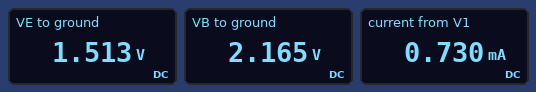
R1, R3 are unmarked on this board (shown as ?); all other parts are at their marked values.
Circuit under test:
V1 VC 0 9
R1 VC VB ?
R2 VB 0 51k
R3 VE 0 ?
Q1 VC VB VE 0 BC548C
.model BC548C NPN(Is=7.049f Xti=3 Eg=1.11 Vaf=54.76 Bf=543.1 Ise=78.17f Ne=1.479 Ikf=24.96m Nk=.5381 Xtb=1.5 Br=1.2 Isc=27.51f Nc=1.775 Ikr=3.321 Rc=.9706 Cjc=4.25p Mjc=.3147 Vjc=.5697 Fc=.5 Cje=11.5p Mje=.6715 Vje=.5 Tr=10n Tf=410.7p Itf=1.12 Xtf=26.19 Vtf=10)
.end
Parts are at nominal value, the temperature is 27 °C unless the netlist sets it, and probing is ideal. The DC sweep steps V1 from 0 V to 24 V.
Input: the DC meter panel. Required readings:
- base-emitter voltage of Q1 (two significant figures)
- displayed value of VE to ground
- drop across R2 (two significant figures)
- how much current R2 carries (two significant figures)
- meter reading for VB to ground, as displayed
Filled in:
650 mV
1.513 V
2.2 V
42 µA
2.165 V
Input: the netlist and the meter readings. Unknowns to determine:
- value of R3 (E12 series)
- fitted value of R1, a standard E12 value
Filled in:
2.2 kΩ
150 kΩ
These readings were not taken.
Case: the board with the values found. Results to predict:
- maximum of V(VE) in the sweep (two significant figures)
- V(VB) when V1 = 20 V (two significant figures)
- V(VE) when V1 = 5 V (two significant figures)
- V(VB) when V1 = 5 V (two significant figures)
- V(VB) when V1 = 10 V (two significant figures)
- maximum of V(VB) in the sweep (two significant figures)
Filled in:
5.1 V
4.8 V
580 mV
1.2 V
2.4 V
5.8 V
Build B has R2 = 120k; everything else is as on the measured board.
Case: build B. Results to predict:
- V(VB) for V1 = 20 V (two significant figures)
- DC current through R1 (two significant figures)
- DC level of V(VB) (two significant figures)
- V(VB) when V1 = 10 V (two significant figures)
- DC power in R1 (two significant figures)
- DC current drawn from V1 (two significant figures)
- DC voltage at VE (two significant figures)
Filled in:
8.1 V
36 µA
3.6 V
4.0 V
190 µW
1.4 mA
3.0 V
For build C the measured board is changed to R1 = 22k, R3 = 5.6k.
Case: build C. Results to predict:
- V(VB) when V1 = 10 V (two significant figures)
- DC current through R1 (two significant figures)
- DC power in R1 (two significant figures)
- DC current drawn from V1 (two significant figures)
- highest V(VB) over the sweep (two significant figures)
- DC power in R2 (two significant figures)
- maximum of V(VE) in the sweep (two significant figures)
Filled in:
6.9 V
130 µA
350 µW
1.1 mA
17 V
760 µW
16 V
